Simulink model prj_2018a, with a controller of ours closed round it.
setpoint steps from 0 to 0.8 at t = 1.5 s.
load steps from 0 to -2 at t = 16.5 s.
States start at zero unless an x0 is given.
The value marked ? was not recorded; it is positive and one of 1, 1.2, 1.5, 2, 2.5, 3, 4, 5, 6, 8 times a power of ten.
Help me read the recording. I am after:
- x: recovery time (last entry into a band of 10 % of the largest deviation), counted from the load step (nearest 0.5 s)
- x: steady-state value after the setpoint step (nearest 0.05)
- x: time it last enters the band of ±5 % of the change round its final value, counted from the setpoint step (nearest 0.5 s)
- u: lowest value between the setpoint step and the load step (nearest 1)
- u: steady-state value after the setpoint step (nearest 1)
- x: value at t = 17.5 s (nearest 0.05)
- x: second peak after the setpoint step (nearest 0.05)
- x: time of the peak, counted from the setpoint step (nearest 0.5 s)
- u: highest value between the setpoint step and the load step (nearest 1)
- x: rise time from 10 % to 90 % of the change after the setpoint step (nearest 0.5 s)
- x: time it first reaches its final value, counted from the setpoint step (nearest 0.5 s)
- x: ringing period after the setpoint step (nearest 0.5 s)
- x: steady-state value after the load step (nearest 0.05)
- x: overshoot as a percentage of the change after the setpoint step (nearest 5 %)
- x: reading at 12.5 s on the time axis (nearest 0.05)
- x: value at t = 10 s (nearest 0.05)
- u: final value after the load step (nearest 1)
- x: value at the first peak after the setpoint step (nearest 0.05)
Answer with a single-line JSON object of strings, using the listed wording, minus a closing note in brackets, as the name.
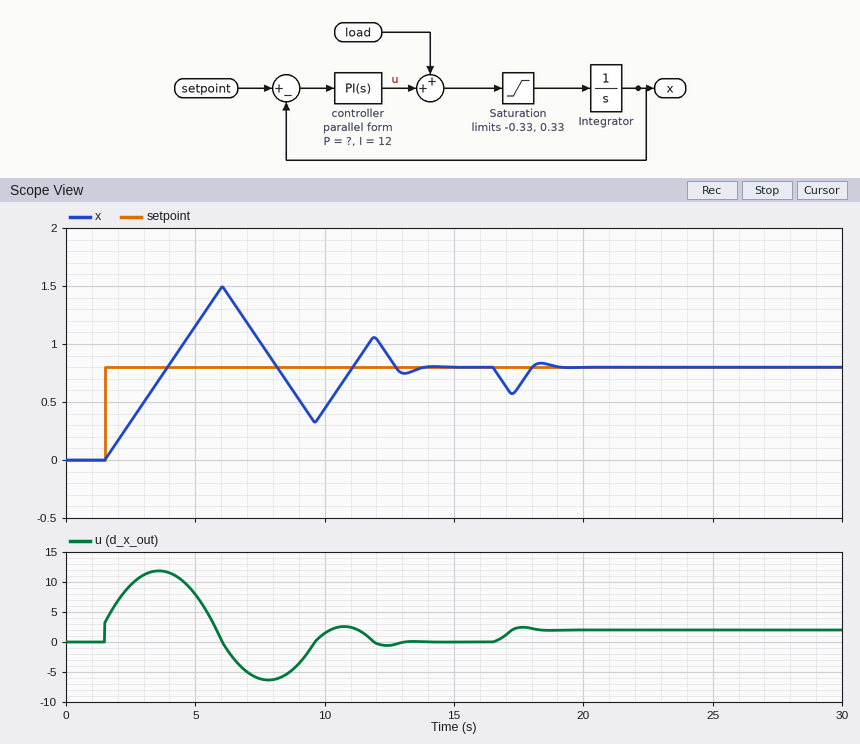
{"x: recovery time (last entry into a band of 10 % of the largest deviation), counted from the load step": "2.0 s", "x: steady-state value after the setpoint step": "0.80", "x: time it last enters the band of ±5 % of the change round its final value, counted from the setpoint step": "12.0 s", "u: lowest value between the setpoint step and the load step": "-6", "u: steady-state value after the setpoint step": "0", "x: value at t = 17.5 s": "0.65", "x: second peak after the setpoint step": "1.05", "x: time of the peak, counted from the setpoint step": "4.5 s", "u: highest value between the setpoint step and the load step": "12", "x: rise time from 10 % to 90 % of the change after the setpoint step": "2.0 s", "x: time it first reaches its final value, counted from the setpoint step": "2.5 s", "x: ringing period after the setpoint step": "6.0 s", "x: steady-state value after the load step": "0.80", "x: overshoot as a percentage of the change after the setpoint step": "85 %", "x: reading at 12.5 s on the time axis": "0.90", "x: value at t = 10 s": "0.45", "u: final value after the load step": "2", "x: value at the first peak after the setpoint step": "1.50"}
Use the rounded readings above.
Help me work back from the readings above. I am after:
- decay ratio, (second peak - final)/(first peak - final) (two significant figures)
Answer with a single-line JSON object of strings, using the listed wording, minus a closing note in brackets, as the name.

{"decay ratio, (second peak - final)/(first peak - final)": "0.36"}
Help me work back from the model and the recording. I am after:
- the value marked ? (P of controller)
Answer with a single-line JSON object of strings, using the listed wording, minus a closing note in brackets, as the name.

{"the value marked ?": "4"}
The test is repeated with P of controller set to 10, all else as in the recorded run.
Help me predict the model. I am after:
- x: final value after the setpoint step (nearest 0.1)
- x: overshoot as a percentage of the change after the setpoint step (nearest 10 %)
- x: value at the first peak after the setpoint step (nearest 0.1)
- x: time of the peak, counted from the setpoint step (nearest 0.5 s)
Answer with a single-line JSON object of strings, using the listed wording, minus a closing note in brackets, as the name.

{"x: final value after the setpoint step": "0.8", "x: overshoot as a percentage of the change after the setpoint step": "70 %", "x: value at the first peak after the setpoint step": "1.4", "x: time of the peak, counted from the setpoint step": "4.0 s"}
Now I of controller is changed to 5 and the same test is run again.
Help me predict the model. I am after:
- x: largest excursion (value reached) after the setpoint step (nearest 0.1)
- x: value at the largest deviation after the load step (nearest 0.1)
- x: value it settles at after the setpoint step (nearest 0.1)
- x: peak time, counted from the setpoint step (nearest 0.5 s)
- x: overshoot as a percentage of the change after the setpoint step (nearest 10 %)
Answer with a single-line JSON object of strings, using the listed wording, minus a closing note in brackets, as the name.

{"x: largest excursion (value reached) after the setpoint step": "1.4", "x: value at the largest deviation after the load step": "0.5", "x: value it settles at after the setpoint step": "0.8", "x: peak time, counted from the setpoint step": "4.0 s", "x: overshoot as a percentage of the change after the setpoint step": "70 %"}
